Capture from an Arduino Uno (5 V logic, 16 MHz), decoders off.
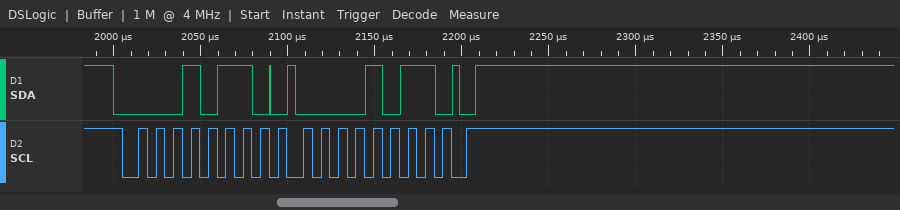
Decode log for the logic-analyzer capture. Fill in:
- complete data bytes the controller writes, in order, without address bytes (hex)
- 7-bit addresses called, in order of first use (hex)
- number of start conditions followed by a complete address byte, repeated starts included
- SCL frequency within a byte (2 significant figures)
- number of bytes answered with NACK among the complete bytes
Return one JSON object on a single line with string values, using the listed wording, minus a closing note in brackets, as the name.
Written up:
{"complete data bytes the controller writes, in order, without address bytes": "0B", "7-bit addresses called, in order of first use": "0x0B", "number of start conditions followed by a complete address byte, repeated starts included": "1", "SCL frequency within a byte": "100 kHz", "number of bytes answered with NACK among the complete bytes": "0"}
